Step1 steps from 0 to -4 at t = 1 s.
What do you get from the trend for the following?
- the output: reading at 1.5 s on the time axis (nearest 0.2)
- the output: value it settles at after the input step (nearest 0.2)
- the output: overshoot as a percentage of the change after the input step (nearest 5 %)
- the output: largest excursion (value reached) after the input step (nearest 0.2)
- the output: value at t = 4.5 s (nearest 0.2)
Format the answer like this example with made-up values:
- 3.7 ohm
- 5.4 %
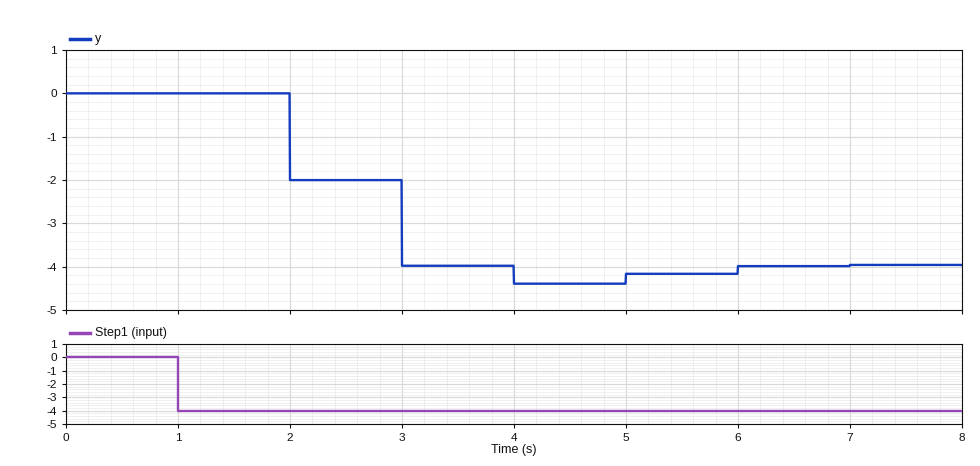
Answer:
- 0.0
- -4.0
- 10 %
- -4.4
- -4.4
